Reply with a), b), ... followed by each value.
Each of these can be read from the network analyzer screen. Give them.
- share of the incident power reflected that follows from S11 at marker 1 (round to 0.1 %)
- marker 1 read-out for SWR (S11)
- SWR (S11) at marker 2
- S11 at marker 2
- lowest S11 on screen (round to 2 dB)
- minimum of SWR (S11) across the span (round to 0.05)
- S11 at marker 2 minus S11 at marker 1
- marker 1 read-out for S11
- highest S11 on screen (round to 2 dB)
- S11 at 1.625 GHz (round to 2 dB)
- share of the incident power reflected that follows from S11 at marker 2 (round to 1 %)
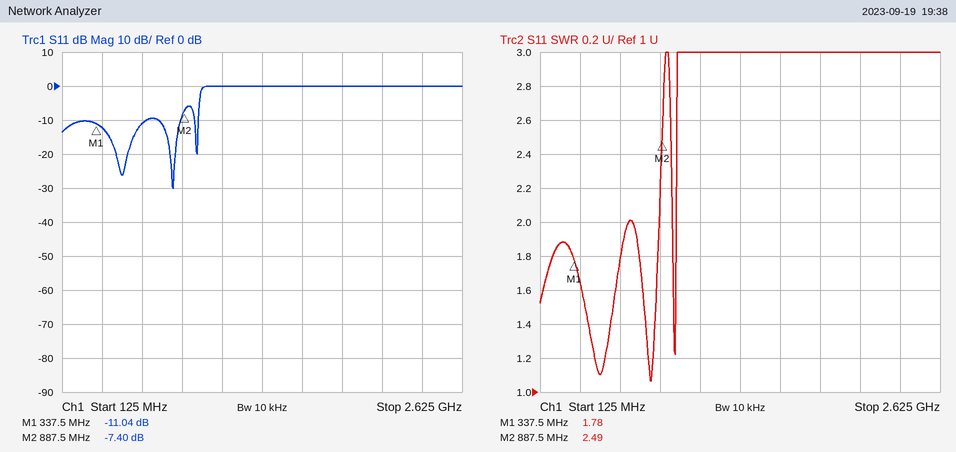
a) 7.9 %
b) 1.78
c) 2.49
d) -7.40 dB
e) -30 dB
f) 1.05
g) 3.64 dB
h) -11.04 dB
i) 0 dB
j) 0 dB
k) 18 %
